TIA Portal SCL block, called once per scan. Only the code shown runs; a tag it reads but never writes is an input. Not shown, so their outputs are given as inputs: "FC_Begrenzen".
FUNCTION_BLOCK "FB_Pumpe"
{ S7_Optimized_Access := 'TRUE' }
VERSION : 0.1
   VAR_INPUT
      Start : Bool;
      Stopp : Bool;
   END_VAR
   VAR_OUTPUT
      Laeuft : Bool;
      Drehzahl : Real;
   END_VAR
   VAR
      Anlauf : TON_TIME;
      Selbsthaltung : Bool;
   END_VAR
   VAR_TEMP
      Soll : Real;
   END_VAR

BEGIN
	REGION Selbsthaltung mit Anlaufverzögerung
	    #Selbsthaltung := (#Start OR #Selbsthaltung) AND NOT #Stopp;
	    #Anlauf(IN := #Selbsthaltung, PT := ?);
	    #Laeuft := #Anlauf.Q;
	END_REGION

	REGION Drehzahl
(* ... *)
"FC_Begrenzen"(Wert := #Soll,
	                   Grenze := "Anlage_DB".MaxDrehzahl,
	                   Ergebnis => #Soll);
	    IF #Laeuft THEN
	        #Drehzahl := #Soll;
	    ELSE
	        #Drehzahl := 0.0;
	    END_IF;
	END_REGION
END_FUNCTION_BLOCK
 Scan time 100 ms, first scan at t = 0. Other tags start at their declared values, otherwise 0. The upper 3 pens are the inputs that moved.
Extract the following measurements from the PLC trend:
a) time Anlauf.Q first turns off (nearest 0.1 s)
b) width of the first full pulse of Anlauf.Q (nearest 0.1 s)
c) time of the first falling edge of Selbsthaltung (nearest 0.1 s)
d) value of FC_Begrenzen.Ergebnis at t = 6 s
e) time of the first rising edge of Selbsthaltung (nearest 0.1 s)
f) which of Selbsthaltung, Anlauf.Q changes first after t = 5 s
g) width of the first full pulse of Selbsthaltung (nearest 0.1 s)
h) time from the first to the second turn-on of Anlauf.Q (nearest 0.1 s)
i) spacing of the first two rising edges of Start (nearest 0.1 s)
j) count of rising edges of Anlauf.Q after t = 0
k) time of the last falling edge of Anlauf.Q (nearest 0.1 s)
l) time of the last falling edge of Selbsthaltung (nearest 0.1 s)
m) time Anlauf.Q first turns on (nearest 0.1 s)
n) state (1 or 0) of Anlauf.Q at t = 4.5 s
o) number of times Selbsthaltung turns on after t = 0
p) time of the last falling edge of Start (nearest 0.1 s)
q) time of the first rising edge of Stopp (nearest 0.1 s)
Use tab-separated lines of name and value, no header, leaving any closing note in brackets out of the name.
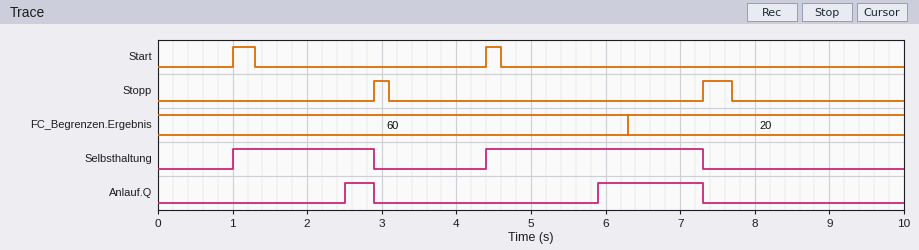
time Anlauf.Q first turns off	2.9 s
width of the first full pulse of Anlauf.Q	0.4 s
time of the first falling edge of Selbsthaltung	2.9 s
value of FC_Begrenzen.Ergebnis at t = 6 s	60
time of the first rising edge of Selbsthaltung	1.0 s
which of Selbsthaltung, Anlauf.Q changes first after t = 5 s	Anlauf.Q
width of the first full pulse of Selbsthaltung	1.9 s
time from the first to the second turn-on of Anlauf.Q	3.4 s
spacing of the first two rising edges of Start	3.4 s
count of rising edges of Anlauf.Q after t = 0	2
time of the last falling edge of Anlauf.Q	7.3 s
time of the last falling edge of Selbsthaltung	7.3 s
time Anlauf.Q first turns on	2.5 s
state (1 or 0) of Anlauf.Q at t = 4.5 s	0
number of times Selbsthaltung turns on after t = 0	2
time of the last falling edge of Start	4.6 s
time of the first rising edge of Stopp	2.9 s
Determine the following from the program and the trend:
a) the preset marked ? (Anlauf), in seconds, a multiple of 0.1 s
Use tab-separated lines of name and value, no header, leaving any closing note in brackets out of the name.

the preset marked ? (Anlauf), in seconds, a multiple of 0.1 s	1.5 s
